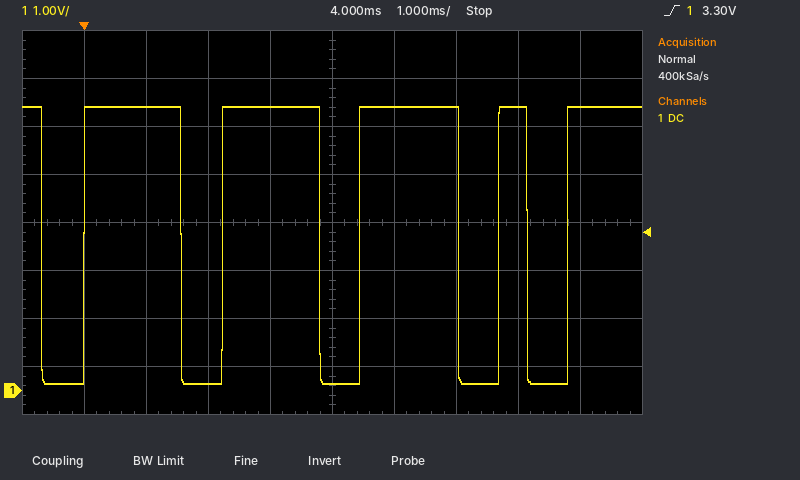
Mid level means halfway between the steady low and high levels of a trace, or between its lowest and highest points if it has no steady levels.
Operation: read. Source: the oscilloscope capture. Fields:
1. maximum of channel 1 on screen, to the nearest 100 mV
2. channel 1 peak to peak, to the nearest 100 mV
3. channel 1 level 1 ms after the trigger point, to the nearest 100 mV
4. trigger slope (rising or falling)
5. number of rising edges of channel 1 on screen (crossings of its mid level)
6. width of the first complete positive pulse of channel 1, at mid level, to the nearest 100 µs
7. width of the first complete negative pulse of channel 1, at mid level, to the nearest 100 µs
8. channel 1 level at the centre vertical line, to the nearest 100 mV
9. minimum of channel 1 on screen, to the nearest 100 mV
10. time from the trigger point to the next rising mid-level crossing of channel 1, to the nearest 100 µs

5.9 V
5.8 V
5.9 V
rising
5
1.6 ms
700 µs
100 mV
100 mV
2.2 ms
